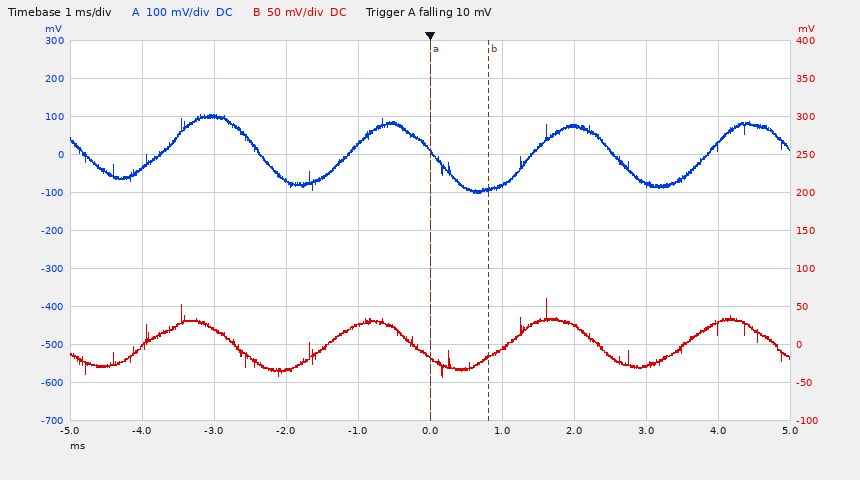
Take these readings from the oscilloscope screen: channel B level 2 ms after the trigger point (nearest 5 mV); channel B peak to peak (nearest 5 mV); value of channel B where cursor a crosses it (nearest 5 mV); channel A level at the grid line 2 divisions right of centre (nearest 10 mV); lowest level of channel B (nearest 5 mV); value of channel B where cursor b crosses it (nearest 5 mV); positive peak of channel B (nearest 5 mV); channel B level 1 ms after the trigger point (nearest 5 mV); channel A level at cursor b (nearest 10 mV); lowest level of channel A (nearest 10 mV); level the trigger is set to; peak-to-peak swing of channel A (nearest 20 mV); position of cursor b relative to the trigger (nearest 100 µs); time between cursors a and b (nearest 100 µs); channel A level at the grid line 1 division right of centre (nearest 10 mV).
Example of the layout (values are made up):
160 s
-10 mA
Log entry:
25 mV
105 mV
-20 mV
70 mV
-45 mV
-15 mV
60 mV
-5 mV
-90 mV
-100 mV
10 mV
200 mV
+800 µs
800 µs
-80 mV
